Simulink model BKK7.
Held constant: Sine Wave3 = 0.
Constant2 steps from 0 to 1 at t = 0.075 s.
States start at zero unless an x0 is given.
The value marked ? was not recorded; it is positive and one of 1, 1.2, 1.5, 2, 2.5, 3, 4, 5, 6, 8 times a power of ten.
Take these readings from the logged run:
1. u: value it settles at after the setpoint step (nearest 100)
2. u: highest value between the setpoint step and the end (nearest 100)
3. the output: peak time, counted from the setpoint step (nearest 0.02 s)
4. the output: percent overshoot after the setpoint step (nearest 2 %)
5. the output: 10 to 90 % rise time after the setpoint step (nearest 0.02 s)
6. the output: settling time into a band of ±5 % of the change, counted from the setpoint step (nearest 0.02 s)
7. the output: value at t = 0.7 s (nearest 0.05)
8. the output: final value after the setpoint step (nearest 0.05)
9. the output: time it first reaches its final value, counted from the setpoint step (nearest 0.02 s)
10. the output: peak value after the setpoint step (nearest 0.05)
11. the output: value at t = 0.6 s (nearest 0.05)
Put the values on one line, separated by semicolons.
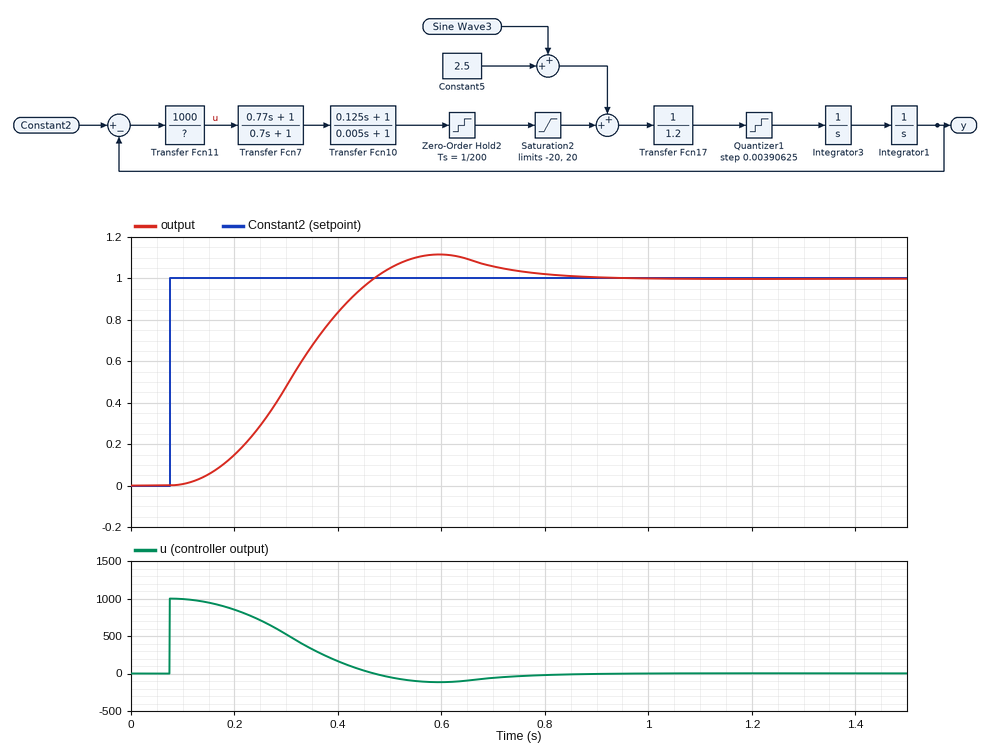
0; 1000; 0.52 s; 12 %; 0.24 s; 0.64 s; 1.05; 1.00; 0.40 s; 1.10; 1.10
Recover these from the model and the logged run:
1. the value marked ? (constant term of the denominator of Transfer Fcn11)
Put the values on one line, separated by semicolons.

1
